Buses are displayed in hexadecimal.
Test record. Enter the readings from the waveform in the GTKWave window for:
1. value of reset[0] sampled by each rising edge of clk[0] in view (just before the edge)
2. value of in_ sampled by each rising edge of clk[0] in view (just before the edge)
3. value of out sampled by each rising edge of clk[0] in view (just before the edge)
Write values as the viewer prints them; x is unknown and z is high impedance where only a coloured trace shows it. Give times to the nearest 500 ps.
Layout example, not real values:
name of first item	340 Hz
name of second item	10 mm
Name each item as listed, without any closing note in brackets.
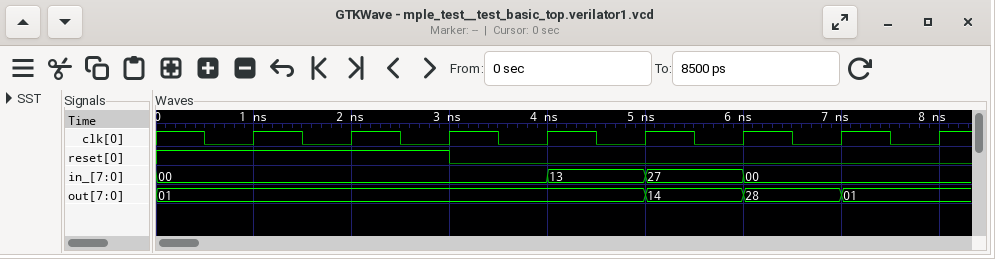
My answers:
value of reset[0] sampled by each rising edge of clk[0] in view	1 1 1 0 0 0 0 0
value of in_ sampled by each rising edge of clk[0] in view	00, 00, 00, 00, 13, 27, 00, 00
value of out sampled by each rising edge of clk[0] in view	01, 01, 01, 01, 01, 14, 28, 01
